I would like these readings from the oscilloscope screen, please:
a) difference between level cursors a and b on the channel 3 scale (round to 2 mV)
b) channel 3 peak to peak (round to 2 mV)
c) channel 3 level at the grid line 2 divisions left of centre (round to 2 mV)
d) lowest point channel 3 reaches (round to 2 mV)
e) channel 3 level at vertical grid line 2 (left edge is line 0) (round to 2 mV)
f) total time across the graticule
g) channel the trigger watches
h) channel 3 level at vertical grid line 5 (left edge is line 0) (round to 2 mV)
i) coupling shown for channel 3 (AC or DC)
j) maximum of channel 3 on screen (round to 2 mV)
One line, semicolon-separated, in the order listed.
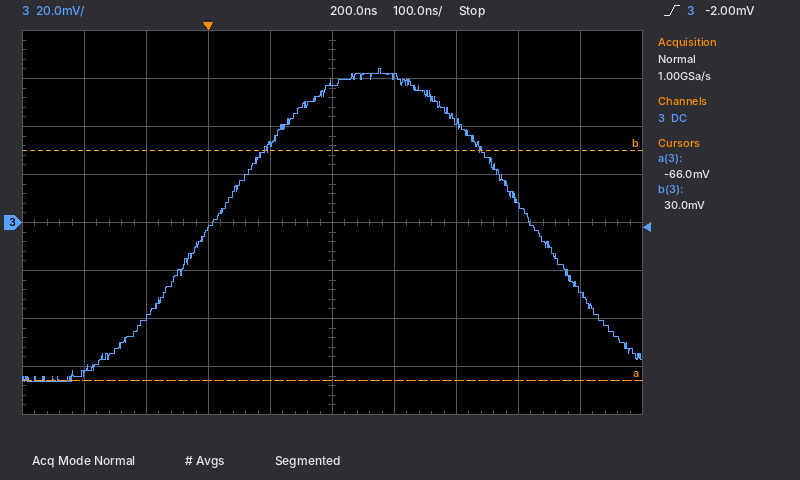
96 mV; 130 mV; -2 mV; -66 mV; -40 mV; 1 µs; channel 3; 58 mV; DC; 64 mV
